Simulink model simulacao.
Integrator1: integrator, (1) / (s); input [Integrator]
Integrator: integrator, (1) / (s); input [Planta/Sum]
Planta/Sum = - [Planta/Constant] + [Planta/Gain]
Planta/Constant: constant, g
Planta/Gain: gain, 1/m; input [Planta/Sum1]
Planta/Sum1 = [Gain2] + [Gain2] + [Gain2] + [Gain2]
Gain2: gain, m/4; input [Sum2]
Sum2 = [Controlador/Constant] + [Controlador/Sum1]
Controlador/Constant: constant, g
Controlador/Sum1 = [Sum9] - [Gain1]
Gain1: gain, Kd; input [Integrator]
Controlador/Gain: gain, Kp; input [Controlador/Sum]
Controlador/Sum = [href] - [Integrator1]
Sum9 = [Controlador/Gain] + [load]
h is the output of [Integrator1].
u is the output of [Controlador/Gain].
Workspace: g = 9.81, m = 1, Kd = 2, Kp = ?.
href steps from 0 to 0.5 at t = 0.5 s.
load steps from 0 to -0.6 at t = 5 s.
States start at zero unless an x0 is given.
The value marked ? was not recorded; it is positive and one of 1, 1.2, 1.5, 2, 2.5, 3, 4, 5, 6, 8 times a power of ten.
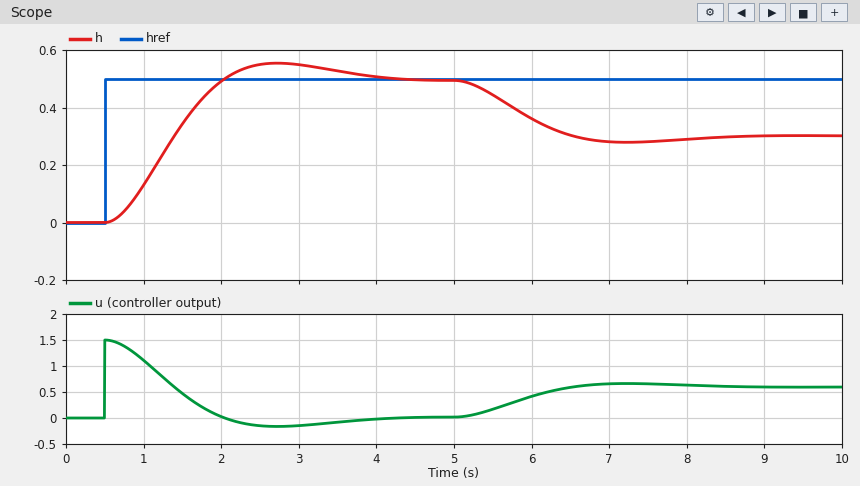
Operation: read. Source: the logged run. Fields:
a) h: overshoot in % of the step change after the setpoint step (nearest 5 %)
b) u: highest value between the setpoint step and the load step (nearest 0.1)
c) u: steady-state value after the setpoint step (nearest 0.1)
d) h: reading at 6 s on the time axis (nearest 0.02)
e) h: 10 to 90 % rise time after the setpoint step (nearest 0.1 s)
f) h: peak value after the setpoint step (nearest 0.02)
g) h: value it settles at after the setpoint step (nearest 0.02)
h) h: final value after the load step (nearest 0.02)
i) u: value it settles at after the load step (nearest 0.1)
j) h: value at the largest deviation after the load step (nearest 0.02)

10 %
1.5
0.0
0.36
1.0 s
0.56
0.50
0.30
0.6
0.28
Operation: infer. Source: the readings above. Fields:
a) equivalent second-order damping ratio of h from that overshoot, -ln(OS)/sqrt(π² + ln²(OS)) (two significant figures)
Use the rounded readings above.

0.59
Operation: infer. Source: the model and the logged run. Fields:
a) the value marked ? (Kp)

3
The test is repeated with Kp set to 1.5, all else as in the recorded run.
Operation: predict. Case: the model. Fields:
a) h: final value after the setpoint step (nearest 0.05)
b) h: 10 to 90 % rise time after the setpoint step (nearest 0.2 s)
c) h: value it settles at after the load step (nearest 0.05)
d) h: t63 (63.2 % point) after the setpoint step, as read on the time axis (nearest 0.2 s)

0.50
2.0 s
0.10
2.0 s
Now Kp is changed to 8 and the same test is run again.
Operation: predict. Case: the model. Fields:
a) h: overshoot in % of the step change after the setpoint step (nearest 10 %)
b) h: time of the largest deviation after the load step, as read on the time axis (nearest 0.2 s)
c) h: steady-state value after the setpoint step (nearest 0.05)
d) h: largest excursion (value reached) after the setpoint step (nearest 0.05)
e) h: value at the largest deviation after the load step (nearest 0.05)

30 %
6.2 s
0.50
0.65
0.40
